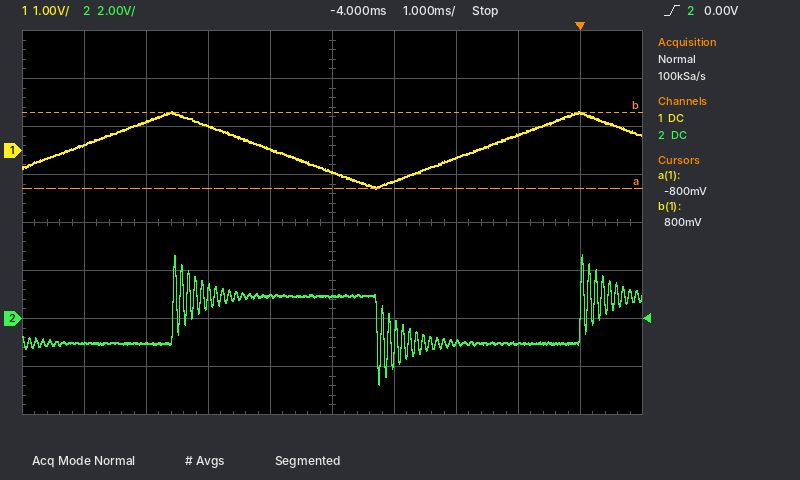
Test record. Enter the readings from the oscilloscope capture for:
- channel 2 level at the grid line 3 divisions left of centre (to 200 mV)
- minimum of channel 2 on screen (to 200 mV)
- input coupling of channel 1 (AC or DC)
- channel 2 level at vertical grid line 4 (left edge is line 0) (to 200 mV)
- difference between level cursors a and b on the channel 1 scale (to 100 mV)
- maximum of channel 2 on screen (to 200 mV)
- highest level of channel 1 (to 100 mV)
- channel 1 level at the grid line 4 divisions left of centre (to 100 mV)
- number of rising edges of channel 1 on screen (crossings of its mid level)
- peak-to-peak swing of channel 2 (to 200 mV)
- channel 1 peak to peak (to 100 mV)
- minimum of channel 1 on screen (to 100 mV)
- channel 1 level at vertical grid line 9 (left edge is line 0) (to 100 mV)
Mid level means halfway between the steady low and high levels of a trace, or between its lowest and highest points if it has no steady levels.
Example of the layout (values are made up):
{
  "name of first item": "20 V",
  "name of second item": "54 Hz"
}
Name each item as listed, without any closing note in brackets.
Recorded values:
{
  "channel 2 level at the grid line 3 divisions left of centre": "-1.0 V",
  "minimum of channel 2 on screen": "-2.8 V",
  "input coupling of channel 1": "DC",
  "channel 2 level at vertical grid line 4 (left edge is line 0)": "1.0 V",
  "difference between level cursors a and b on the channel 1 scale": "1.6 V",
  "maximum of channel 2 on screen": "2.6 V",
  "highest level of channel 1": "800 mV",
  "channel 1 level at the grid line 4 divisions left of centre": "100 mV",
  "number of rising edges of channel 1 on screen": "2",
  "peak-to-peak swing of channel 2": "5.4 V",
  "channel 1 peak to peak": "1.6 V",
  "minimum of channel 1 on screen": "-800 mV",
  "channel 1 level at vertical grid line 9 (left edge is line 0)": "800 mV"
}
